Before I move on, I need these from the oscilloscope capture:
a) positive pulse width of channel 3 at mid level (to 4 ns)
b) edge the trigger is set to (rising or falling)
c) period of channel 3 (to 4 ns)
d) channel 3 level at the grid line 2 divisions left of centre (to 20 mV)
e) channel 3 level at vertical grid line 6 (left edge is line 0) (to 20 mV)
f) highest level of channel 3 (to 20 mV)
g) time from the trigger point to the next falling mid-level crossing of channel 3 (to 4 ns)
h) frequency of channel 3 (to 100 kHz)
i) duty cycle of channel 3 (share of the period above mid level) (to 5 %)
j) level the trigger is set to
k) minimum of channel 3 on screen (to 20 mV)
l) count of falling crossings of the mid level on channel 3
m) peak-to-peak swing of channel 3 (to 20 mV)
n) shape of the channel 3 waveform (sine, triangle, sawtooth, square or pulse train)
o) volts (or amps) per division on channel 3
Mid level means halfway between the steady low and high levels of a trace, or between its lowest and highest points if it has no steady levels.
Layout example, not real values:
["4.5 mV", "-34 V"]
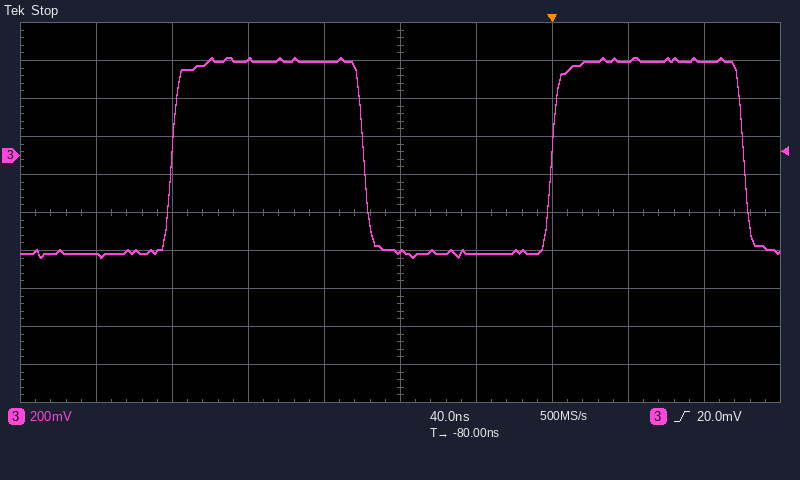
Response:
["100 ns", "rising", "200 ns", "500 mV", "-520 mV", "520 mV", "100 ns", "5.0 MHz", "50 %", "20.0 mV", "-540 mV", "2", "1.06 V", "square", "200 mV"]
